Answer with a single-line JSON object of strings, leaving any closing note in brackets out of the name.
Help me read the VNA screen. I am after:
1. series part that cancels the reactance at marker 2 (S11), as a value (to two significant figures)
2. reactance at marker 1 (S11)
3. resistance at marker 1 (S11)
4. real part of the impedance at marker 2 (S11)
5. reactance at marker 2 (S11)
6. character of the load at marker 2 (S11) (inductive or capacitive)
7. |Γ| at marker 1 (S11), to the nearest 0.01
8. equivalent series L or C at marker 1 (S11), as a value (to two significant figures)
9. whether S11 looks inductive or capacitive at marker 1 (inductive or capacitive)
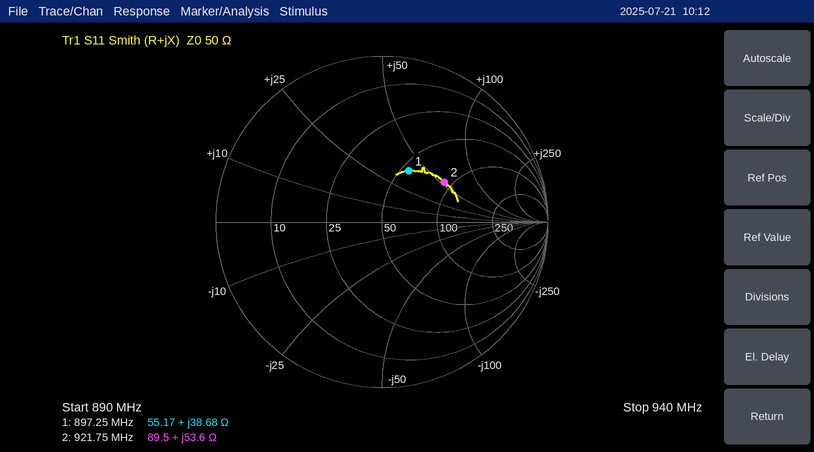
{"series part that cancels the reactance at marker 2 (S11), as a value": "3.2 pF", "reactance at marker 1": "+38.68 Ω", "resistance at marker 1": "55.17 Ω", "real part of the impedance at marker 2": "89.5 Ω", "reactance at marker 2": "+53.6 Ω", "character of the load at marker 2 (S11)": "inductive", "|Γ| at marker 1 (S11), to the nearest 0.01": "0.35", "equivalent series L or C at marker 1 (S11), as a value": "6.9 nH", "whether S11 looks inductive or capacitive at marker 1": "inductive"}
